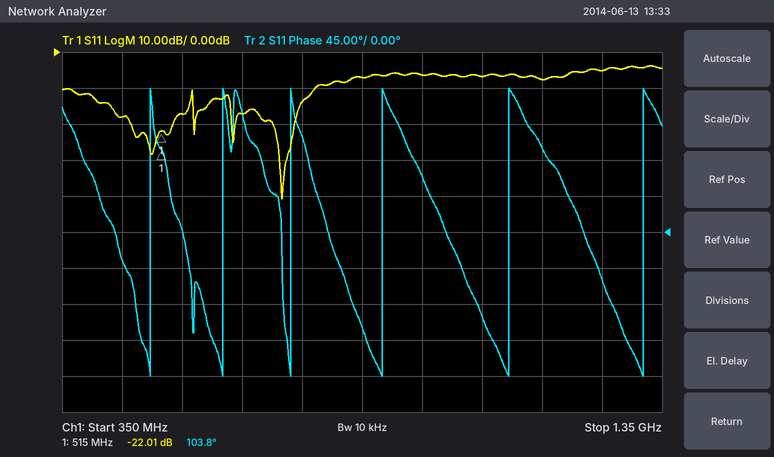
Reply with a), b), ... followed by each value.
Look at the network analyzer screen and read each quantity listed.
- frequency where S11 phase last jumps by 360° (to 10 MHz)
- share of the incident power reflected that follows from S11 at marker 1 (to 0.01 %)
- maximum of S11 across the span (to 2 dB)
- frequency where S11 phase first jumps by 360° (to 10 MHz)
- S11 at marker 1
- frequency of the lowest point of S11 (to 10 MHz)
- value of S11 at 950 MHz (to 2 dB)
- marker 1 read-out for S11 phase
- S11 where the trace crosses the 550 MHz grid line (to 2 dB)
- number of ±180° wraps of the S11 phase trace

a) 1.32 GHz
b) 0.63 %
c) -4 dB
d) 500 MHz
e) -22.01 dB
f) 720 MHz
g) -6 dB
h) 103.8°
i) -18 dB
j) 6
